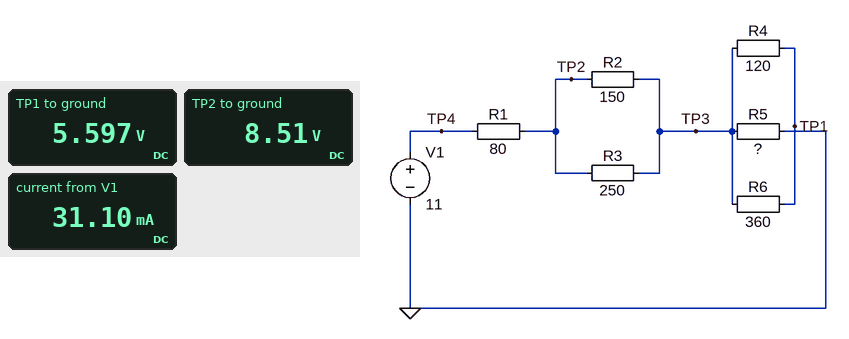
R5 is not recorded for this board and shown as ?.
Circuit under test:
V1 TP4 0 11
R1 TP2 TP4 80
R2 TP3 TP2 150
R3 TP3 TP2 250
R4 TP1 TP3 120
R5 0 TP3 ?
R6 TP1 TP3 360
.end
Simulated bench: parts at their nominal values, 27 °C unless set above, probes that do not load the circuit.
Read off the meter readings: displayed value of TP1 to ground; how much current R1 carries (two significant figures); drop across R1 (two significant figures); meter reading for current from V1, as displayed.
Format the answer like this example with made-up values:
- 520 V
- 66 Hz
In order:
- 5.597 V
- 31 mA
- 2.5 V
- 31.10 mA
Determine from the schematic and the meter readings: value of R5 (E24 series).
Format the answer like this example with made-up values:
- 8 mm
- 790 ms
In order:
- 180 Ω
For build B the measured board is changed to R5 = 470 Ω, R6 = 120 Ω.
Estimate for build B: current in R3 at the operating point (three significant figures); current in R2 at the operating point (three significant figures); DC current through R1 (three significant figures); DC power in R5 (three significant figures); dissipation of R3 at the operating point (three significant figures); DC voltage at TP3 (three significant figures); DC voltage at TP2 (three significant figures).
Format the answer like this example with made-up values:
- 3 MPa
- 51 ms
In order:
- 6.41 mA
- 10.7 mA
- 17.1 mA
- 137 mW
- 10.3 mW
- 8.03 V
- 9.63 V
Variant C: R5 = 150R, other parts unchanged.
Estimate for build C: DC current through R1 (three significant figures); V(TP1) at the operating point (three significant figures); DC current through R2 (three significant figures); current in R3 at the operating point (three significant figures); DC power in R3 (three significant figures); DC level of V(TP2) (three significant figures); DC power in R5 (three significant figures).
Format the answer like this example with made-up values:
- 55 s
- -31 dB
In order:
- 34.0 mA
- 5.10 V
- 21.2 mA
- 12.7 mA
- 40.6 mW
- 8.28 V
- 173 mW
